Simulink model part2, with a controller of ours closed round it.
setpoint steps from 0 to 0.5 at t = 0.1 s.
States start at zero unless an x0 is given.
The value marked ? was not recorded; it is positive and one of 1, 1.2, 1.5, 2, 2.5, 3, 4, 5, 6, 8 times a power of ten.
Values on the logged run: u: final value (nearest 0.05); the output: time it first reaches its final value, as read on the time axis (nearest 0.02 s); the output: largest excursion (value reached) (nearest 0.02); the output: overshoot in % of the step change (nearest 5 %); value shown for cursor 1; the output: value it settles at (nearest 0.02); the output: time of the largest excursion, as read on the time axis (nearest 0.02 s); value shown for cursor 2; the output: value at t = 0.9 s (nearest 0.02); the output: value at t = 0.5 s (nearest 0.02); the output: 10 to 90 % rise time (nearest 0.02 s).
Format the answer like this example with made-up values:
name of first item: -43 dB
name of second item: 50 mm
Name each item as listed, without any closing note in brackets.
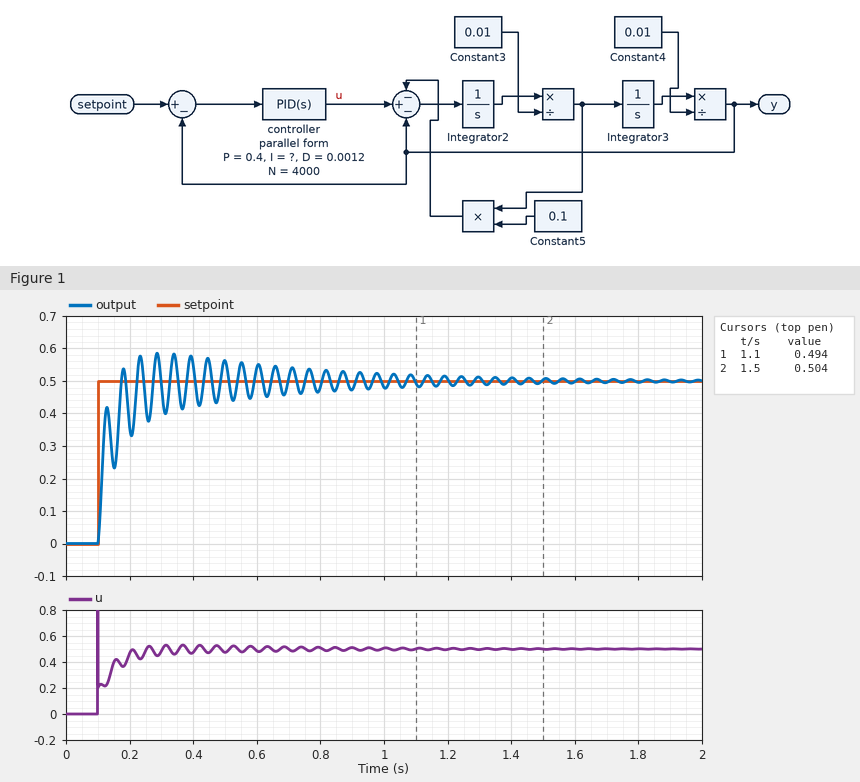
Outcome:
u: final value: 0.50
the output: time it first reaches its final value, as read on the time axis: 0.18 s
the output: largest excursion (value reached): 0.58
the output: overshoot in % of the step change: 15 %
value shown for cursor 1: 0.494
the output: value it settles at: 0.50
the output: time of the largest excursion, as read on the time axis: 0.28 s
value shown for cursor 2: 0.504
the output: value at t = 0.9 s: 0.48
the output: value at t = 0.5 s: 0.56
the output: 10 to 90 % rise time: 0.06 s
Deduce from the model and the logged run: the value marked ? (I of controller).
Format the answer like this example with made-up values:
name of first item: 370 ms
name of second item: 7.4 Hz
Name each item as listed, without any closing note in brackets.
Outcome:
the value marked ?: 25
